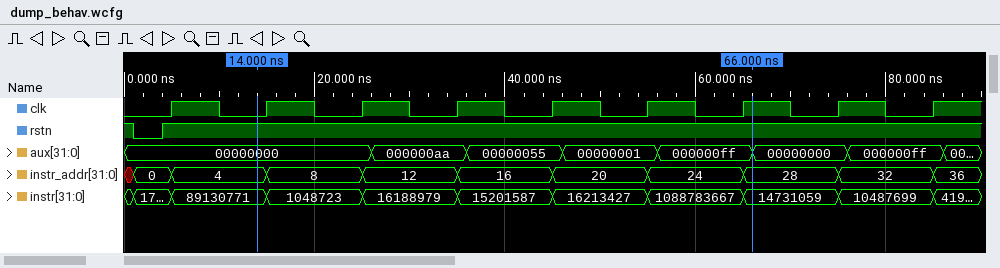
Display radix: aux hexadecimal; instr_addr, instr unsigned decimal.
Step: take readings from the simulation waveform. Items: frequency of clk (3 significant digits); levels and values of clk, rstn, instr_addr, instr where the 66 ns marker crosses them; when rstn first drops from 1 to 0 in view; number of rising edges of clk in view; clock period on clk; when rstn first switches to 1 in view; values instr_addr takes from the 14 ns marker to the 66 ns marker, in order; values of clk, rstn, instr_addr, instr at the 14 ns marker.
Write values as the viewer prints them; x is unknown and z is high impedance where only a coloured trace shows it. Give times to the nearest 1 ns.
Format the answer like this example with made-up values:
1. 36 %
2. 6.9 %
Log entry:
1. 100 MHz
2. clk=1, rstn=1, instr_addr=28, instr=14731059
3. 1 ns
4. 9
5. 10 ns
6. 4 ns
7. 4, 8, 12, 16, 20, 24, 28
8. clk=0, rstn=1, instr_addr=4, instr=89130771
